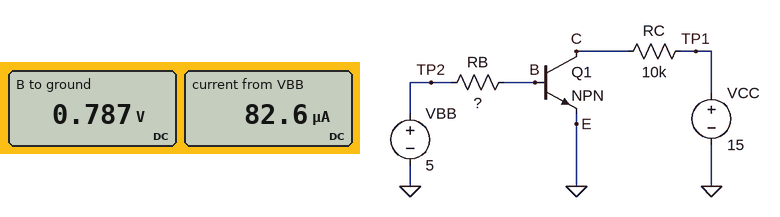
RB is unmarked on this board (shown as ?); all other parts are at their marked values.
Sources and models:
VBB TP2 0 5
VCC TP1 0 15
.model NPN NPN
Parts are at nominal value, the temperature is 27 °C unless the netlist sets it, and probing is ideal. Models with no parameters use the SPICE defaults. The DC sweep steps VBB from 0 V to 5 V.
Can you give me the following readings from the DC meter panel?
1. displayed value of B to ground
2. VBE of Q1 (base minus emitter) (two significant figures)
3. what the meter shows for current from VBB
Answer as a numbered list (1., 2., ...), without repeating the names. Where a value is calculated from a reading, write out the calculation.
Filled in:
1. 0.787 V
2. 787 mV = 790 mV
3. 82.6 µA
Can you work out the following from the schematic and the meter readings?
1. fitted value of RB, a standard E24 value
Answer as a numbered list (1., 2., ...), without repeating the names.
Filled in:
1. 51 kΩ
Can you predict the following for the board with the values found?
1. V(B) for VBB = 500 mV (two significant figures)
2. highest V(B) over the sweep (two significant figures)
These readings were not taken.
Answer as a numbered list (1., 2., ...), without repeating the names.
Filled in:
1. 500 mV
2. 790 mV
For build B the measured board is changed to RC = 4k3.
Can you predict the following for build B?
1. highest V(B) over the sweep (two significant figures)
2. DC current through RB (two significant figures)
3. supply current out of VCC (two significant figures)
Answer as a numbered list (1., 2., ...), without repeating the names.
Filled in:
1. 810 mV
2. 82 µA
3. 3.5 mA
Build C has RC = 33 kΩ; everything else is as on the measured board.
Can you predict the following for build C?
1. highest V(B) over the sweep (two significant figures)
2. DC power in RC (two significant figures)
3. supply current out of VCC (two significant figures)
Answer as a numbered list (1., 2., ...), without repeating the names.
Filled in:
1. 760 mV
2. 6.8 mW
3. 450 µA
